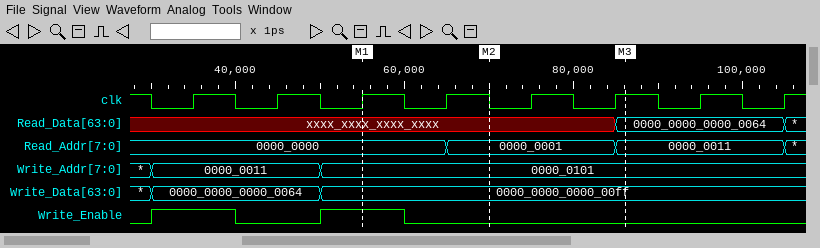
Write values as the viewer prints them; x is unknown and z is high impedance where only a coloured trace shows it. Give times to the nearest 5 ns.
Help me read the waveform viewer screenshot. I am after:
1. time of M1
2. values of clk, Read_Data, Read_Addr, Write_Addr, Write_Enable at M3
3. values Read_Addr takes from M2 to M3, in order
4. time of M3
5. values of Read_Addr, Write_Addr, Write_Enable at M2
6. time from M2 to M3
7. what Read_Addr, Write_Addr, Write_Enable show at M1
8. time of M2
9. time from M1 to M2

55 ns
clk=1, Read_Data=0000_0000_0000_0064, Read_Addr=0000_0011, Write_Addr=0000_0101, Write_Enable=0
0000_0001, 0000_0011
85 ns
Read_Addr=0000_0001, Write_Addr=0000_0101, Write_Enable=0
15 ns
Read_Addr=0000_0000, Write_Addr=0000_0101, Write_Enable=1
70 ns
15 ns
